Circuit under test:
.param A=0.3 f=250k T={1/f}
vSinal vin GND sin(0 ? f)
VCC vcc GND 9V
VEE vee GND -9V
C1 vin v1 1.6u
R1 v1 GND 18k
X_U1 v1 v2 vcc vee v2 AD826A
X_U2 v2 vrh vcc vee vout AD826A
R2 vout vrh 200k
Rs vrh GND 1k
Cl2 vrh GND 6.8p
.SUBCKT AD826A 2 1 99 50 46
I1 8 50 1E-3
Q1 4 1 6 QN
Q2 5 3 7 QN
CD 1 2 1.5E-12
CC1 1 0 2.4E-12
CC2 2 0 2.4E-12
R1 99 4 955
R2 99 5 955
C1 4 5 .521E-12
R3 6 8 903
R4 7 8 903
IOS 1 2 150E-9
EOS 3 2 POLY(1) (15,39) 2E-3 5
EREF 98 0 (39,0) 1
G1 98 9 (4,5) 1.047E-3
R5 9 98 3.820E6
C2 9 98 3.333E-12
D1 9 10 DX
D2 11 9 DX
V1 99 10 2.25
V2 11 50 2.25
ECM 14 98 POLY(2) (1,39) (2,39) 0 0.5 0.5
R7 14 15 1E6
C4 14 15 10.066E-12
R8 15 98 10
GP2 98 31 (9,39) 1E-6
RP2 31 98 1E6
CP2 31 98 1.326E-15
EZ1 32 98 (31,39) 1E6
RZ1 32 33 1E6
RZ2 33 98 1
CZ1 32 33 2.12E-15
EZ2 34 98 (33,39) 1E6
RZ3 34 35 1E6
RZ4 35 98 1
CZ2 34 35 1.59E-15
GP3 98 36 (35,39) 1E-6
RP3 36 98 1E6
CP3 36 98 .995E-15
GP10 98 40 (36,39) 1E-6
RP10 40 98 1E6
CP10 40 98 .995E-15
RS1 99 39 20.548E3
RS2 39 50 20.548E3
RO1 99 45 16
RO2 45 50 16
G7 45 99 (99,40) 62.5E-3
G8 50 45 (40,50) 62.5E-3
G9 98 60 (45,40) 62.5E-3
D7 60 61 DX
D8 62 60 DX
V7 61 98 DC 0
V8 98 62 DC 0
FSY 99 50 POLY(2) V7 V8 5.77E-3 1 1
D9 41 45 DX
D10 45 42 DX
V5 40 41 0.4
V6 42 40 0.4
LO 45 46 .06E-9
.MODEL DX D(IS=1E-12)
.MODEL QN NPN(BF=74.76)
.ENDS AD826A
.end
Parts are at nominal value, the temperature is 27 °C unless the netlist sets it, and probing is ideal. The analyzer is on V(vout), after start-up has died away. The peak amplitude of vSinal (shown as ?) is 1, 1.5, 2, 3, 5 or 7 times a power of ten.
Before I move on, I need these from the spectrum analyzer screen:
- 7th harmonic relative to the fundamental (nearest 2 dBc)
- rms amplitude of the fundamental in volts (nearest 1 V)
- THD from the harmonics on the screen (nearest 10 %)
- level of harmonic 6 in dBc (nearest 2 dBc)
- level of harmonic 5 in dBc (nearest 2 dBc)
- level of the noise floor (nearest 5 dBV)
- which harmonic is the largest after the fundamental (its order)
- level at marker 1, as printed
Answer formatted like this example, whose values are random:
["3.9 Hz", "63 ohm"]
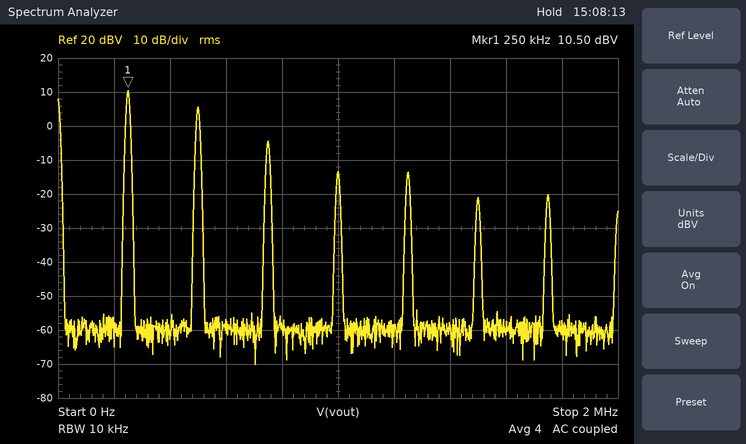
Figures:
["-30 dBc", "3 V", "60 %", "-32 dBc", "-24 dBc", "-60 dBV", "2", "10.50 dBV"]
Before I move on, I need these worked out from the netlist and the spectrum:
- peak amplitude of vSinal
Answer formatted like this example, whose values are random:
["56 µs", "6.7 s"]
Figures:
["150 mV"]
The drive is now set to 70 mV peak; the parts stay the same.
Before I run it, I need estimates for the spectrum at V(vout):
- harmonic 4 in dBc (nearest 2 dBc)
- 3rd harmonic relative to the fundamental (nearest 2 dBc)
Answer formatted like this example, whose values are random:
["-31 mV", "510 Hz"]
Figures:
["-10 dBc", "-8 dBc"]
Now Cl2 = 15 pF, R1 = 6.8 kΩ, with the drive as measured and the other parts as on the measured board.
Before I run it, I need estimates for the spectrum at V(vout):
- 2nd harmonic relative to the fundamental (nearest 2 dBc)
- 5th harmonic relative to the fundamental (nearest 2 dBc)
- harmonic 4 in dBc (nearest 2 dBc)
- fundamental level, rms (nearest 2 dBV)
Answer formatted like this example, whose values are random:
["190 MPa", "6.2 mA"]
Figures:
["-14 dBc", "-34 dBc", "-20 dBc", "16 dBV"]
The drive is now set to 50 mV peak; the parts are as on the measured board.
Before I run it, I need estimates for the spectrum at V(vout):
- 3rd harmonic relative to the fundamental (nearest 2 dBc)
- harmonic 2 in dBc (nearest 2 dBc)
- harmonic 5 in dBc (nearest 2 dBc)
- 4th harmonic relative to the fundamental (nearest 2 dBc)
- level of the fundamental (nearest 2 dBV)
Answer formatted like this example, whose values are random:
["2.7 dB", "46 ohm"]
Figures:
["-24 dBc", "-14 dBc", "-42 dBc", "-34 dBc", "-36 dBV"]
